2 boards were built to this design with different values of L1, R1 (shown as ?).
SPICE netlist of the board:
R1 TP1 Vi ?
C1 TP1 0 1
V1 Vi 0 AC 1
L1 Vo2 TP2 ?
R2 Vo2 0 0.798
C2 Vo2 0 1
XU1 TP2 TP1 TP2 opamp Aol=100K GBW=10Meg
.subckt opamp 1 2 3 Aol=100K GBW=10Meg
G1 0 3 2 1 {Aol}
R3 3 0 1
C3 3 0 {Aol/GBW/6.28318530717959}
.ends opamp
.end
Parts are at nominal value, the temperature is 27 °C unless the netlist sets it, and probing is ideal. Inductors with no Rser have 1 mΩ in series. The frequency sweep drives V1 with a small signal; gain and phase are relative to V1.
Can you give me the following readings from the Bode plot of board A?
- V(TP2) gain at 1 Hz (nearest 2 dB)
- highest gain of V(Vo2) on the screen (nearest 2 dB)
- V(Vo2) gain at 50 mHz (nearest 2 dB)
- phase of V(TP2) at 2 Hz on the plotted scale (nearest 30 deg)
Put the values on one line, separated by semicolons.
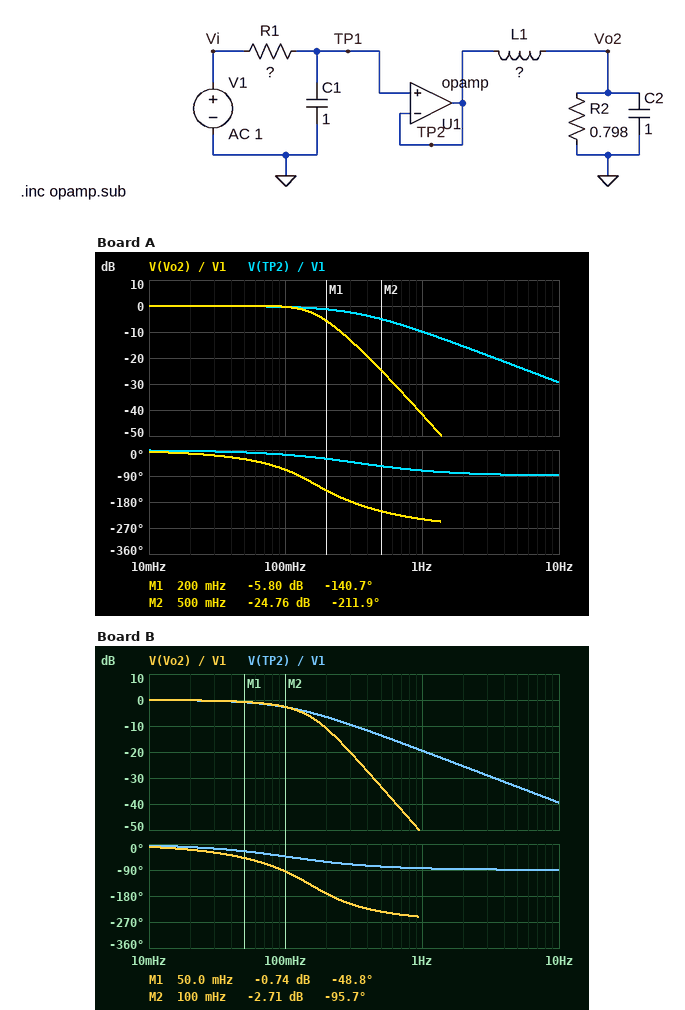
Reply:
-10 dB; 0 dB; 0 dB; -90 deg
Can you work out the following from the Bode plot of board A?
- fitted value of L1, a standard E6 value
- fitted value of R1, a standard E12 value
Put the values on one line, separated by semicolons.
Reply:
1 H; 0.47 Ω
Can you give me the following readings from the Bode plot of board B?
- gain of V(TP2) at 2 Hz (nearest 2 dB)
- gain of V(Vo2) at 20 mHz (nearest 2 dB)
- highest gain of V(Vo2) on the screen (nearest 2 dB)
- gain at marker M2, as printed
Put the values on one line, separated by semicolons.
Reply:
-26 dB; 0 dB; 0 dB; -2.71 dB
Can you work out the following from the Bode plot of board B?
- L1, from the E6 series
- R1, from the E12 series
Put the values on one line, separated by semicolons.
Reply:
1 H; 1.5 Ω
